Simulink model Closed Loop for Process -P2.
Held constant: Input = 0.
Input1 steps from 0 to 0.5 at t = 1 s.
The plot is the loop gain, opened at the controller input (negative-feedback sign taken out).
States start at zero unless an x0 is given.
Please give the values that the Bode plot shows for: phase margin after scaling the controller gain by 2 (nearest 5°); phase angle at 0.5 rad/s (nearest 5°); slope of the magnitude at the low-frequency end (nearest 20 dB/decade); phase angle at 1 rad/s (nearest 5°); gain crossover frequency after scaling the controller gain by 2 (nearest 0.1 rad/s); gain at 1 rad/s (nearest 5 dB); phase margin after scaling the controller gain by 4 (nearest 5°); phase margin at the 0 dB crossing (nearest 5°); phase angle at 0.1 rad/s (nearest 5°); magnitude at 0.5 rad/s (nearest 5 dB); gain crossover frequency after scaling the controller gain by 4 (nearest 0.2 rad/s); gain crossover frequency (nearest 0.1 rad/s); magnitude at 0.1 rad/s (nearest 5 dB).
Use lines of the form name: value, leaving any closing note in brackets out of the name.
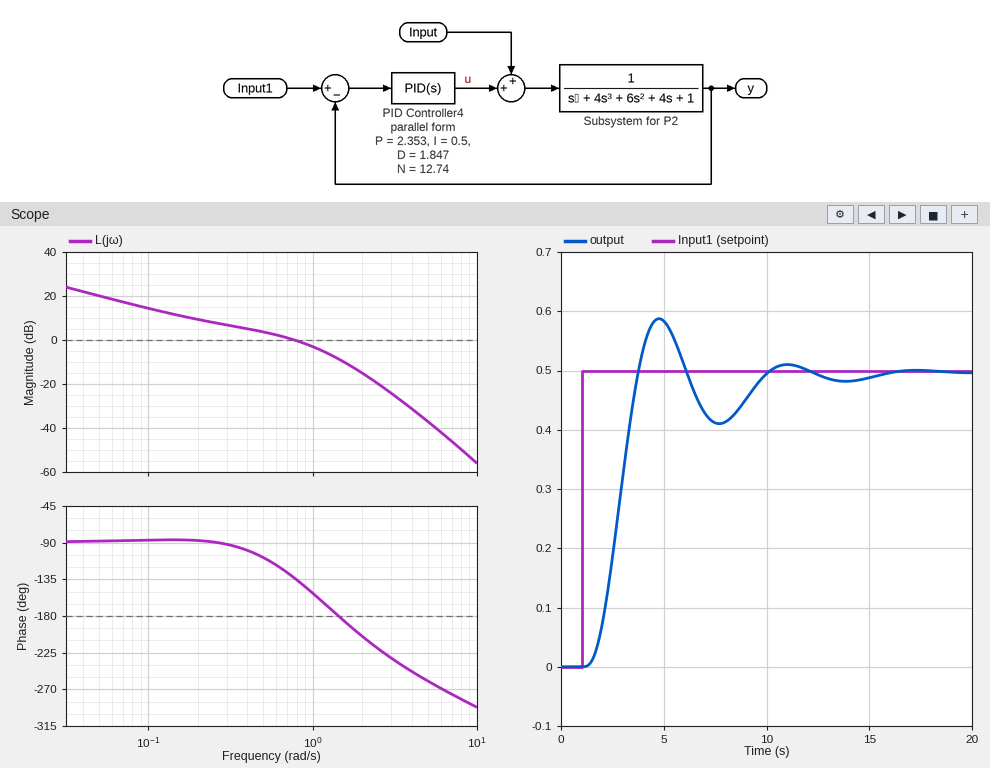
phase margin after scaling the controller gain by 2: 10°
phase angle at 0.5 rad/s: -110°
slope of the magnitude at the low-frequency end: -20 dB/decade
phase angle at 1 rad/s: -150°
gain crossover frequency after scaling the controller gain by 2: 1.2 rad/s
gain at 1 rad/s: -5 dB
phase margin after scaling the controller gain by 4: -15°
phase margin at the 0 dB crossing: 45°
phase angle at 0.1 rad/s: -85°
magnitude at 0.5 rad/s: 5 dB
gain crossover frequency after scaling the controller gain by 4: 1.8 rad/s
gain crossover frequency: 0.8 rad/s
magnitude at 0.1 rad/s: 15 dB
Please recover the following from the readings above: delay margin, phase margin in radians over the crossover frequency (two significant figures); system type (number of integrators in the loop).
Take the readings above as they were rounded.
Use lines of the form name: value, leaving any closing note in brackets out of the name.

delay margin, phase margin in radians over the crossover frequency: 0.98 s
system type: 1
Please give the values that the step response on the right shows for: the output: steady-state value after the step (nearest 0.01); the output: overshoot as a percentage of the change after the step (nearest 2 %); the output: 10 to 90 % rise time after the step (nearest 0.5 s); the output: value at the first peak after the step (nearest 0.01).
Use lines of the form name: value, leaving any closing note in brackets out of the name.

the output: steady-state value after the step: 0.50
the output: overshoot as a percentage of the change after the step: 18 %
the output: 10 to 90 % rise time after the step: 1.5 s
the output: value at the first peak after the step: 0.59
